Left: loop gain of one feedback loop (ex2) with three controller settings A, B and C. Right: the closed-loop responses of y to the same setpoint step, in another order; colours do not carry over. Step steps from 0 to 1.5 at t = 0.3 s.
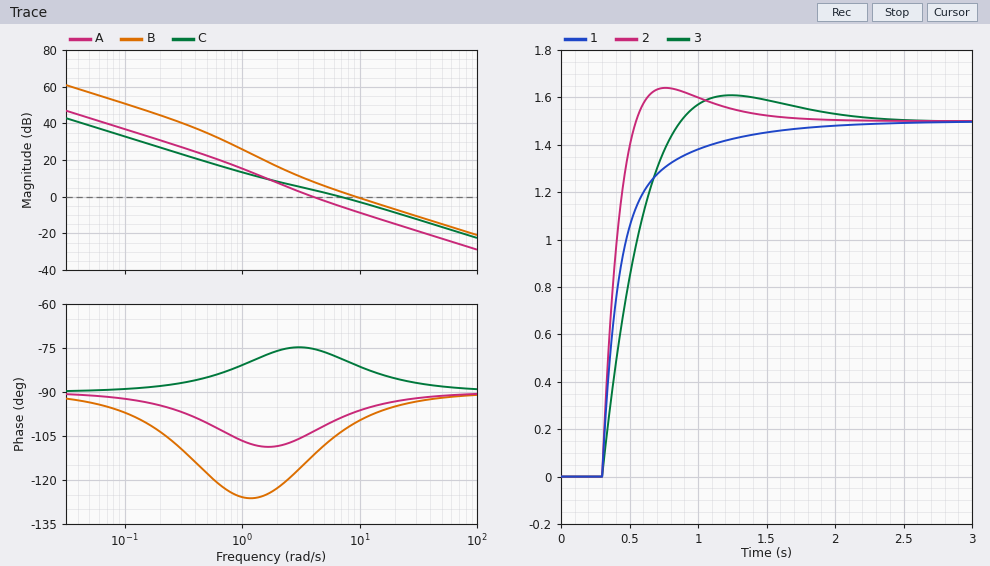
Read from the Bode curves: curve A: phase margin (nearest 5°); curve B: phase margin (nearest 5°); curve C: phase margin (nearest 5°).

75°
80°
100°
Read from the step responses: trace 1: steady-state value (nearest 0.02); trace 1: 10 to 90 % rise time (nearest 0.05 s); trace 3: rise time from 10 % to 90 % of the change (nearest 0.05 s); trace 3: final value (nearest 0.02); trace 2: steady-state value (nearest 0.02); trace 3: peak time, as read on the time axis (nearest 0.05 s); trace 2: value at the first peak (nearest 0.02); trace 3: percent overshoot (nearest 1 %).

1.50
0.55 s
0.40 s
1.50
1.50
1.25 s
1.64
7 %
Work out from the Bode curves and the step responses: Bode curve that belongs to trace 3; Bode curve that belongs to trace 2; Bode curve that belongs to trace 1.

A
B
C
